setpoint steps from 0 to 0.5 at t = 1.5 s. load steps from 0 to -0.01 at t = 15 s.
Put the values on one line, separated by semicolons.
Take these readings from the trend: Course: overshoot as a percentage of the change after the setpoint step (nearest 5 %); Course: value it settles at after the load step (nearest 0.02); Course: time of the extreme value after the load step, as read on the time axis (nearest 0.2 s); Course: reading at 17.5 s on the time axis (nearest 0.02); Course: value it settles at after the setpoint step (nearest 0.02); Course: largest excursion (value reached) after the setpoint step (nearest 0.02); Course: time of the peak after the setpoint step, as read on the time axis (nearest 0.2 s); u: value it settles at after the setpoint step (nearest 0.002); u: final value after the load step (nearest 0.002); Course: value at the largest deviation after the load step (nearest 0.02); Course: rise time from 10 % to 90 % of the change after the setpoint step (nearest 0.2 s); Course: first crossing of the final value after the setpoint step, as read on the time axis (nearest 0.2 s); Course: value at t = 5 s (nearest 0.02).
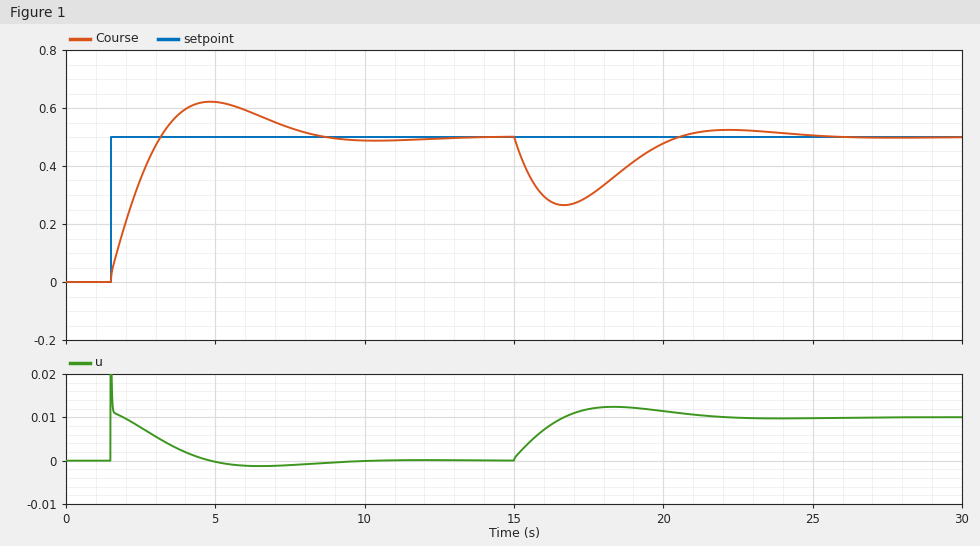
25 %; 0.50; 16.6 s; 0.30; 0.50; 0.62; 4.8 s; 0.000; 0.010; 0.26; 1.4 s; 3.2 s; 0.62
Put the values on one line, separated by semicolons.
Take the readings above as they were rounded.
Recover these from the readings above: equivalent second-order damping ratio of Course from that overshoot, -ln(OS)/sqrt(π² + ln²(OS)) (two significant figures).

0.40
